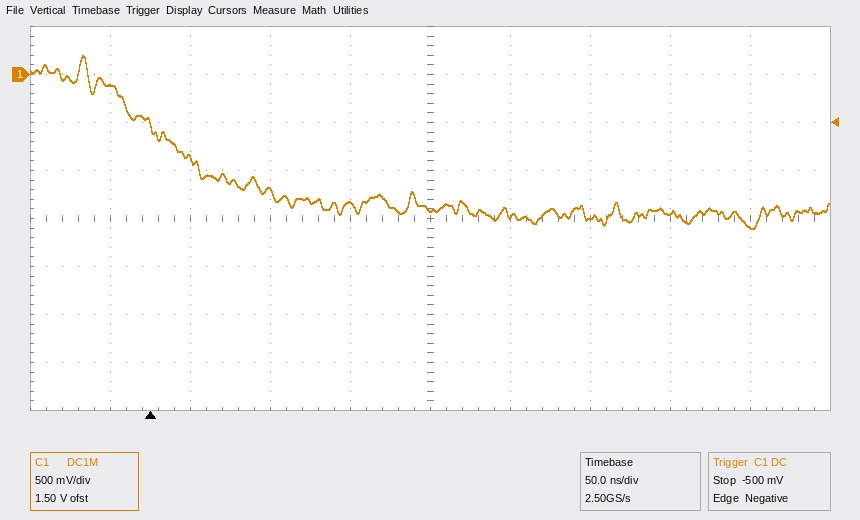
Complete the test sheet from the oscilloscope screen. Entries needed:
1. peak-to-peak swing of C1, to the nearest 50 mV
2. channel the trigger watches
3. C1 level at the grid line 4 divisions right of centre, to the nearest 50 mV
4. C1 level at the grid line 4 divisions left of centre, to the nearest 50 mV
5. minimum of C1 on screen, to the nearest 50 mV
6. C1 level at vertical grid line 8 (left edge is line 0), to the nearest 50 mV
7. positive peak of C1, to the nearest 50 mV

1.80 V
C1
-1.60 V
-100 mV
-1.60 V
-1.45 V
200 mV
